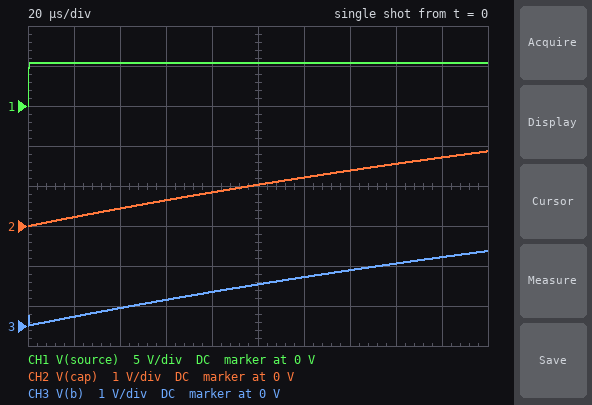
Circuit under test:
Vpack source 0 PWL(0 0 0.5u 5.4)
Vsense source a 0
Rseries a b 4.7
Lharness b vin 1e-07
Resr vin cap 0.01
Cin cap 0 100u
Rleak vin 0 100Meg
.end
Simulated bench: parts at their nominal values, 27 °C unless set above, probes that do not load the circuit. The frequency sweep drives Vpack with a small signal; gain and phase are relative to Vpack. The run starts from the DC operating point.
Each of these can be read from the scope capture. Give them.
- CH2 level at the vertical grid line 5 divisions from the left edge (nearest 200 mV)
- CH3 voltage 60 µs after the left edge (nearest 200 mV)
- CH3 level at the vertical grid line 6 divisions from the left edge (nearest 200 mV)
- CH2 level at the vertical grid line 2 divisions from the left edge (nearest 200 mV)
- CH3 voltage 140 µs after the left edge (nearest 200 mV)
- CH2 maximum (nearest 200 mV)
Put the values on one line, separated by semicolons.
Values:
1.0 V; 600 mV; 1.2 V; 400 mV; 1.4 V; 1.8 V
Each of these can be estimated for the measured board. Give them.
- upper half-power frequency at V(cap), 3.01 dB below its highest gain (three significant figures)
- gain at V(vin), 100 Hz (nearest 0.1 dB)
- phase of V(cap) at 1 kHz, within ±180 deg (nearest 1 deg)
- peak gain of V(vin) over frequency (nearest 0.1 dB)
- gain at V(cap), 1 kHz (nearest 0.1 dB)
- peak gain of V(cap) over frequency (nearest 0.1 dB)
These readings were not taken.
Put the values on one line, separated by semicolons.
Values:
338 Hz; -0.4 dB; -71 deg; 0 dB; -9.9 dB; 0 dB
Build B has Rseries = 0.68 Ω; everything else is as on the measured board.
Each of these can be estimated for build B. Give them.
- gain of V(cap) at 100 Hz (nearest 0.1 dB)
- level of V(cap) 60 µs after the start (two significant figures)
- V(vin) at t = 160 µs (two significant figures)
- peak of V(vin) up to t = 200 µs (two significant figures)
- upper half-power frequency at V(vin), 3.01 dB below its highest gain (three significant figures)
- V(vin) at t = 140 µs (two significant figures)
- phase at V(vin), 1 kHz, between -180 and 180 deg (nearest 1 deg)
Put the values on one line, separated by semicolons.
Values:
0 dB; 3.1 V; 4.9 V; 5.1 V; 2.31 kHz; 4.7 V; -23 deg
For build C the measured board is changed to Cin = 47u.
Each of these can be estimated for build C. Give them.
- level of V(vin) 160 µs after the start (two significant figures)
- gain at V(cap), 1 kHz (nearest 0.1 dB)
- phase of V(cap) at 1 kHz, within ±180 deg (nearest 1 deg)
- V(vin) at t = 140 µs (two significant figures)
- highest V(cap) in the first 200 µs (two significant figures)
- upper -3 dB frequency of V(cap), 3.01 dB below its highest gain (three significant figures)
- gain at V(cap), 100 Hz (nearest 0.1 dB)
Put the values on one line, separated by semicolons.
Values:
2.8 V; -4.7 dB; -54 deg; 2.5 V; 3.2 V; 719 Hz; -0.1 dB
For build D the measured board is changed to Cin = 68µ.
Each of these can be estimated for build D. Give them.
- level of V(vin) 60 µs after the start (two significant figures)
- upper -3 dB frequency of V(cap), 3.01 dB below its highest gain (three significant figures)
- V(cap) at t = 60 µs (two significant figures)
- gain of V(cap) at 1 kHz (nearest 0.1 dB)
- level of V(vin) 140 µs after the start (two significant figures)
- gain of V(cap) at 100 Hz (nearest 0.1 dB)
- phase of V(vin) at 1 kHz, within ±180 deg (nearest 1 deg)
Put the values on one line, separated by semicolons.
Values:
930 mV; 497 Hz; 920 mV; -7.0 dB; 1.9 V; -0.2 dB; -63 deg
